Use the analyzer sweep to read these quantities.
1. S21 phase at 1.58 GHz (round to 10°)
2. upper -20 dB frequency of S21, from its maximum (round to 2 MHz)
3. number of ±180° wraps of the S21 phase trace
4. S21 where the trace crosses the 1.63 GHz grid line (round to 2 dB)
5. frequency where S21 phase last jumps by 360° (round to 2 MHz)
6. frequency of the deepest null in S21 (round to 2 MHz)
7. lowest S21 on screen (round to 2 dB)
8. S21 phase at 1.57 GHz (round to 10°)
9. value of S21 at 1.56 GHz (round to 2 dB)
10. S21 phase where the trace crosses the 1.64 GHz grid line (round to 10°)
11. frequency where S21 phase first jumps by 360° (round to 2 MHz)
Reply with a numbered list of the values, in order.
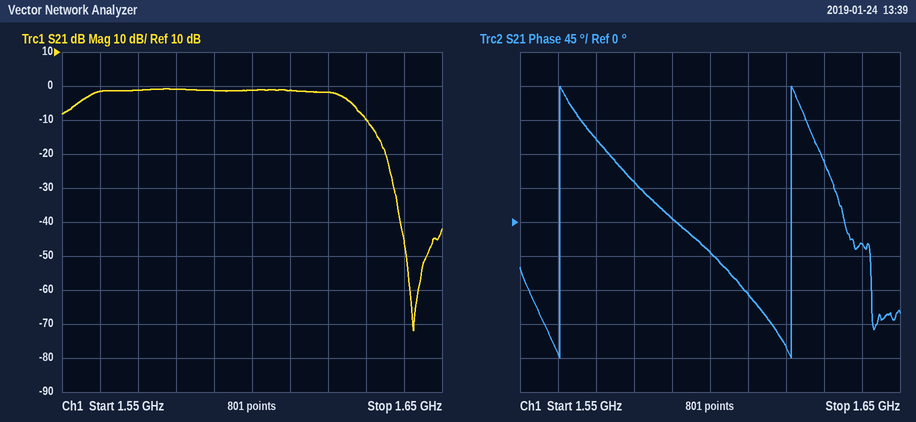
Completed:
1. 50°
2. 1.636 GHz
3. 2
4. -10 dB
5. 1.622 GHz
6. 1.642 GHz
7. -72 dB
8. 110°
9. -2 dB
10. -30°
11. 1.560 GHz
